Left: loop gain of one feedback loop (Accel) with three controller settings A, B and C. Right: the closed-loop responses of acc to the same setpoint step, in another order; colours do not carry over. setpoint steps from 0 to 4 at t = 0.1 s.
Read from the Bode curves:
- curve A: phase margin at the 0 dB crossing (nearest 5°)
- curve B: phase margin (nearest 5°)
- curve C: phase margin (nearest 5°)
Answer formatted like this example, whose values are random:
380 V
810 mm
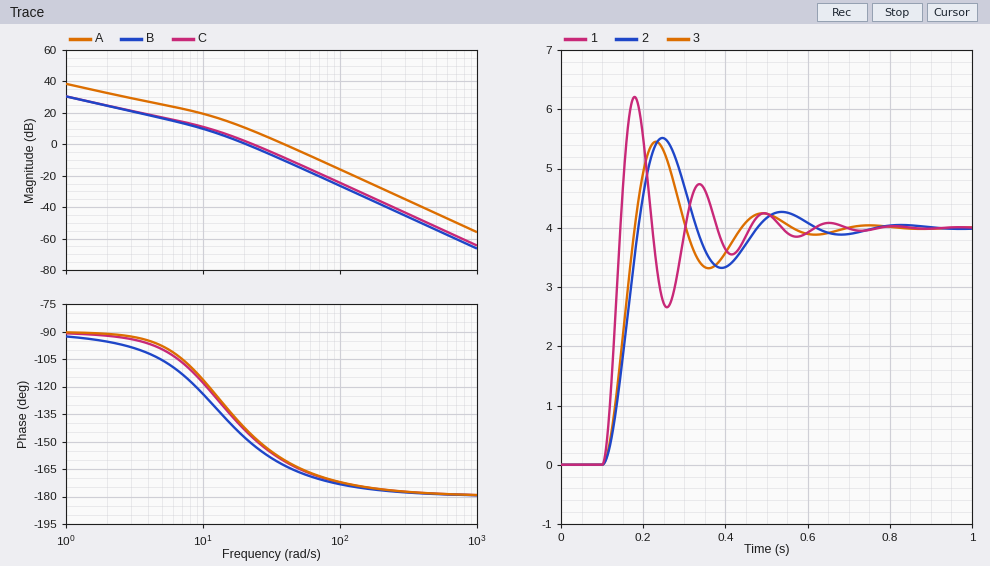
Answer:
20°
30°
30°
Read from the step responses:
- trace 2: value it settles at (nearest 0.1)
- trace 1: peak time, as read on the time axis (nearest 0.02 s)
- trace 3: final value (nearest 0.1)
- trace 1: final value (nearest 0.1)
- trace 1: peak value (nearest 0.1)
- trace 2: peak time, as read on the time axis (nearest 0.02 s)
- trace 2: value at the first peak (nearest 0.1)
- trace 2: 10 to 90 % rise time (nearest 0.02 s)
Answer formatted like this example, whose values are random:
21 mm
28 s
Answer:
4.0
0.18 s
4.0
4.0
6.2
0.24 s
5.5
0.06 s
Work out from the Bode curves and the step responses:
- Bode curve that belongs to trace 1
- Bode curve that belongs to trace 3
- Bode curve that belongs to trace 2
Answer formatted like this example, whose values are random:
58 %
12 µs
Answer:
A
C
B
